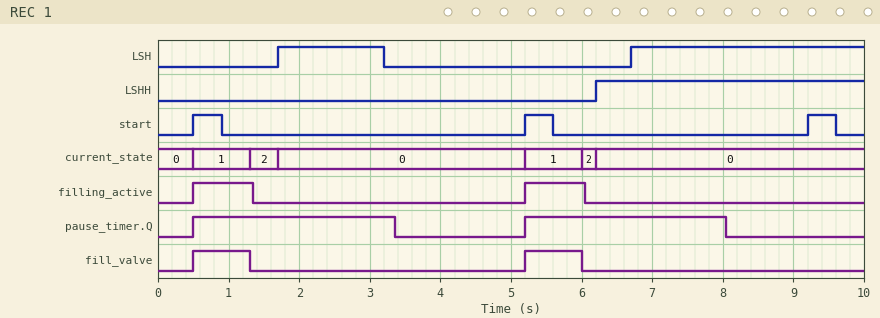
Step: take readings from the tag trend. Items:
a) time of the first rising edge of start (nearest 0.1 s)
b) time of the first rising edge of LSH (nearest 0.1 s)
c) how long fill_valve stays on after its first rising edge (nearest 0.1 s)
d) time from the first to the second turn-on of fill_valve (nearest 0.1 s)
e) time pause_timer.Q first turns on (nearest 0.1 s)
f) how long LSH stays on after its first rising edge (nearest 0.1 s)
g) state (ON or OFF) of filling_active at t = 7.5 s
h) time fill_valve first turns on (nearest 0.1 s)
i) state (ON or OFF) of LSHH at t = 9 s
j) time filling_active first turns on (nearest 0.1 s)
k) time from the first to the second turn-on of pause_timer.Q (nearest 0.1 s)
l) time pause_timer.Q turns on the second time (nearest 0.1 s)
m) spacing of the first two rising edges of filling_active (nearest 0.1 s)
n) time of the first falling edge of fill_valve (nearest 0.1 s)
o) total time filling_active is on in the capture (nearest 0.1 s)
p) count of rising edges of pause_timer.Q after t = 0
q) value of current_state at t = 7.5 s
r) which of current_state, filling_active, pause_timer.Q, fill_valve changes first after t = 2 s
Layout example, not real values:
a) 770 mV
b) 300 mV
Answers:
a) 0.5 s
b) 1.7 s
c) 0.8 s
d) 4.7 s
e) 0.5 s
f) 1.5 s
g) OFF
h) 0.5 s
i) ON
j) 0.5 s
k) 4.7 s
l) 5.2 s
m) 4.7 s
n) 1.3 s
o) 1.7 s
p) 2
q) 0
r) pause_timer.Q
